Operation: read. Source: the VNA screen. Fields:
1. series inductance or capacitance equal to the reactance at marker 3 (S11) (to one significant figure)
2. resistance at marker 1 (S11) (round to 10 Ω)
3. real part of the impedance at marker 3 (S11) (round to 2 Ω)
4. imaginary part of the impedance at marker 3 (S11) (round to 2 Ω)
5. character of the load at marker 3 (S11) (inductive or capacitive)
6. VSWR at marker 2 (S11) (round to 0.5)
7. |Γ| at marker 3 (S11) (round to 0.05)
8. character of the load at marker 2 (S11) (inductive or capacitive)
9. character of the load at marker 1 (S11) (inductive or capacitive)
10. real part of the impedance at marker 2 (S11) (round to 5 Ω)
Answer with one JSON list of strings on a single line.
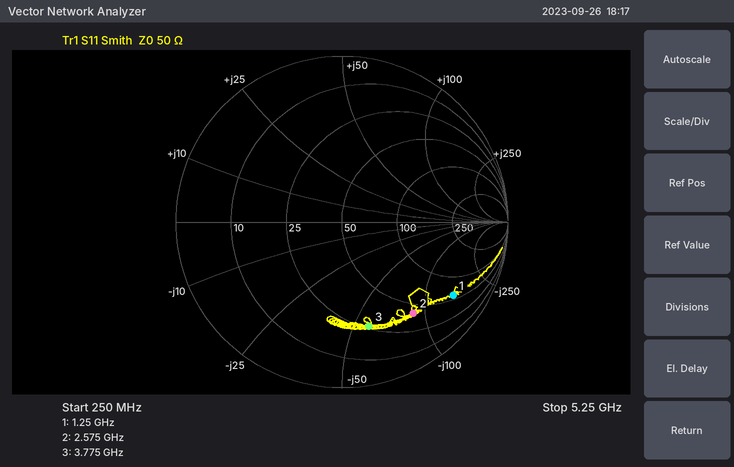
["700 fF", "60 Ω", "26 Ω", "-58 Ω", "capacitive", "5.5", "0.65", "capacitive", "capacitive", "40 Ω"]
